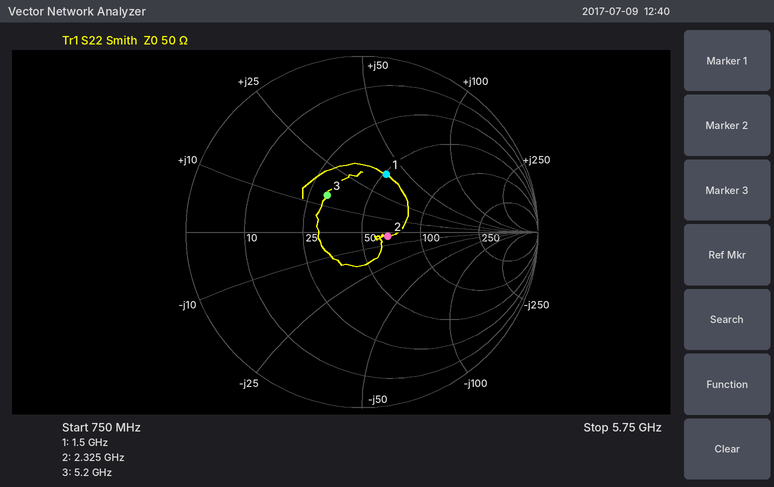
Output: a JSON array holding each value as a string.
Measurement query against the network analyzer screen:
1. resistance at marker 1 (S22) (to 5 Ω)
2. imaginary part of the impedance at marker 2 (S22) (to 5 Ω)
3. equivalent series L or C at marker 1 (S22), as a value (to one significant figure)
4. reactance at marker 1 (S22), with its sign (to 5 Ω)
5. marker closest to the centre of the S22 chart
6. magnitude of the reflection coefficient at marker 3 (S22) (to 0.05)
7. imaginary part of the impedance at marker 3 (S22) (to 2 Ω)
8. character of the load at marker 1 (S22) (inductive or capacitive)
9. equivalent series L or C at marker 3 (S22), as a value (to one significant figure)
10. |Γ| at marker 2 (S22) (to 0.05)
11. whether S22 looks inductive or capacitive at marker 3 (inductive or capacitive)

["50 Ω", "-5 Ω", "4 nH", "+40 Ω", "marker 2", "0.30", "+14 Ω", "inductive", "400 pH", "0.15", "inductive"]
